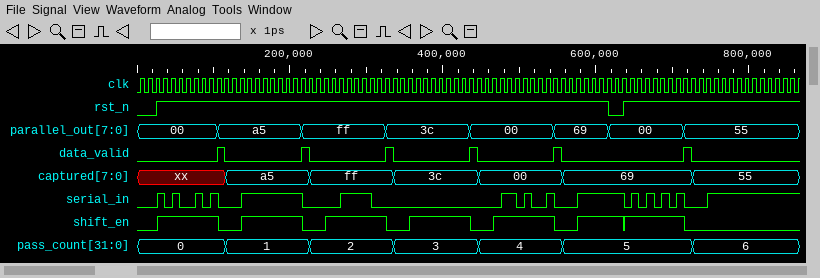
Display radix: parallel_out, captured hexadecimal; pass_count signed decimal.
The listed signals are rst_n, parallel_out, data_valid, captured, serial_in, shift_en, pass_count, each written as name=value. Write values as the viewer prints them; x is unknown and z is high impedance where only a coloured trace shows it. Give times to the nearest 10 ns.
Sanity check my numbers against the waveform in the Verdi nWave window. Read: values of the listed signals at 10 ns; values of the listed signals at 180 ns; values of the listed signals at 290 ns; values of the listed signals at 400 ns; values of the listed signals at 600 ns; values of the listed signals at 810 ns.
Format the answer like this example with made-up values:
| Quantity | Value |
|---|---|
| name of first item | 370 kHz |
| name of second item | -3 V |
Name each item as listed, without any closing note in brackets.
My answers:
| Quantity | Value |
|---|---|
| values of the listed signals at 10 ns | rst_n=0, parallel_out=00, data_valid=0, captured=xx, serial_in=0, shift_en=0, pass_count=0 |
| values of the listed signals at 180 ns | rst_n=1, parallel_out=a5, data_valid=0, captured=a5, serial_in=1, shift_en=1, pass_count=1 |
| values of the listed signals at 290 ns | rst_n=1, parallel_out=ff, data_valid=0, captured=ff, serial_in=1, shift_en=1, pass_count=2 |
| values of the listed signals at 400 ns | rst_n=1, parallel_out=3c, data_valid=0, captured=3c, serial_in=0, shift_en=1, pass_count=3 |
| values of the listed signals at 600 ns | rst_n=1, parallel_out=69, data_valid=0, captured=69, serial_in=1, shift_en=1, pass_count=5 |
| values of the listed signals at 810 ns | rst_n=1, parallel_out=55, data_valid=0, captured=55, serial_in=1, shift_en=0, pass_count=6 |
